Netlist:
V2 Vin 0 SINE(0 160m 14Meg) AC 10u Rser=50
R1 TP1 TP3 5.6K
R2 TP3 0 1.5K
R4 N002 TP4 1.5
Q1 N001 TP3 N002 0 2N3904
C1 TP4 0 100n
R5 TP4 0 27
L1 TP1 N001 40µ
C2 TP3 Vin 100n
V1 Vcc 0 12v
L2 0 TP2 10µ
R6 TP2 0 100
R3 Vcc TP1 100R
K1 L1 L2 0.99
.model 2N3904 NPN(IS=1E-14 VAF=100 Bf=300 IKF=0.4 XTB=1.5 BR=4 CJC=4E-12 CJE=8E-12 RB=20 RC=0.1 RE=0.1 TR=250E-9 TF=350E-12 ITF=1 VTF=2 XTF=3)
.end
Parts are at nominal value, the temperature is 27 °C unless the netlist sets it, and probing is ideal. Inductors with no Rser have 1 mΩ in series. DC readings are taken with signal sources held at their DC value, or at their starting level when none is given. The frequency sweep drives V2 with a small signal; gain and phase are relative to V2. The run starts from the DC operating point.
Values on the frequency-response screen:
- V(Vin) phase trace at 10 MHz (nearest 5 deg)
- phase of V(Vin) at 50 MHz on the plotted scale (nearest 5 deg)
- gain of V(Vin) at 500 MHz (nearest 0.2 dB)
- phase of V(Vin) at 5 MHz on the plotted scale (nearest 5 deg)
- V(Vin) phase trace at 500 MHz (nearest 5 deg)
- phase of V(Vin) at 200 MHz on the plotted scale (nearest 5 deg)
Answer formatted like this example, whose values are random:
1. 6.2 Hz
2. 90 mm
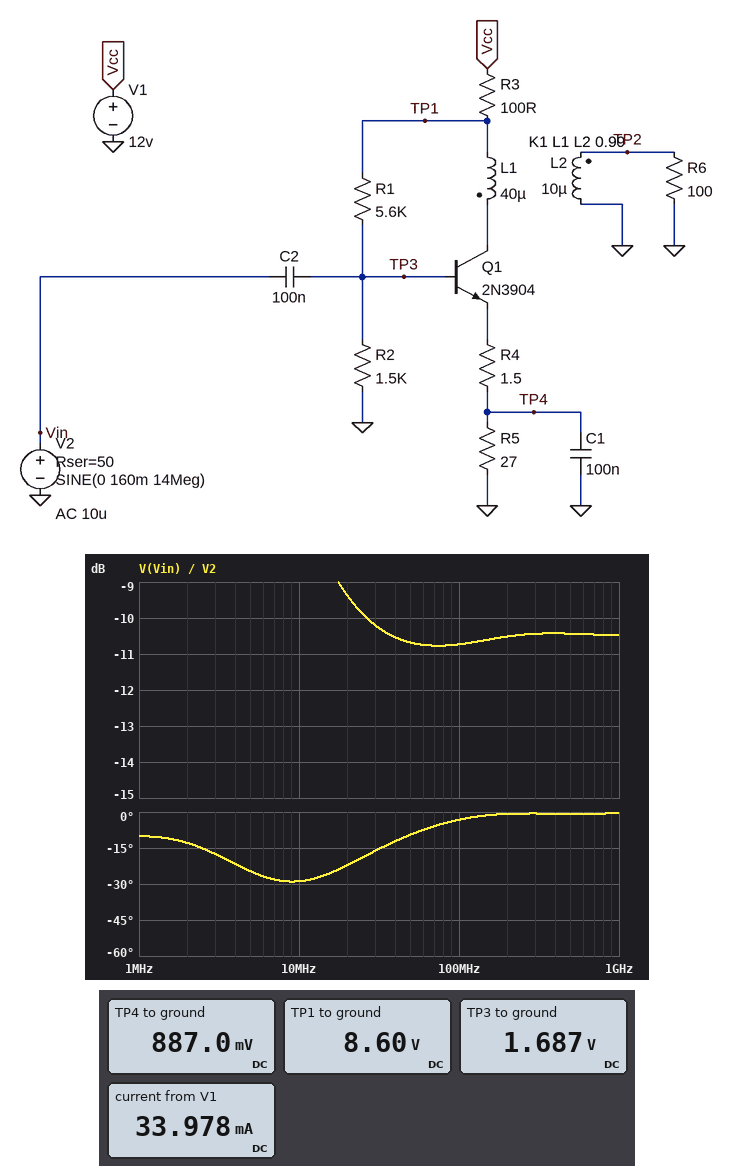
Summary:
1. -30 deg
2. -10 deg
3. -10.4 dB
4. -25 deg
5. 0 deg
6. 0 deg
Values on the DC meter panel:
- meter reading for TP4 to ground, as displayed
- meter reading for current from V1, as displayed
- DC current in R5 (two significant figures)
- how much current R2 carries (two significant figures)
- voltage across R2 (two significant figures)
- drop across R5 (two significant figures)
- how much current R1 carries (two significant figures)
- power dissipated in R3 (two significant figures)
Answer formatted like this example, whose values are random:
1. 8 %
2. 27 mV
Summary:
1. 887.0 mV
2. 33.978 mA
3. 33 mA
4. 1.1 mA
5. 1.7 V
6. 890 mV
7. 1.2 mA
8. 120 mW
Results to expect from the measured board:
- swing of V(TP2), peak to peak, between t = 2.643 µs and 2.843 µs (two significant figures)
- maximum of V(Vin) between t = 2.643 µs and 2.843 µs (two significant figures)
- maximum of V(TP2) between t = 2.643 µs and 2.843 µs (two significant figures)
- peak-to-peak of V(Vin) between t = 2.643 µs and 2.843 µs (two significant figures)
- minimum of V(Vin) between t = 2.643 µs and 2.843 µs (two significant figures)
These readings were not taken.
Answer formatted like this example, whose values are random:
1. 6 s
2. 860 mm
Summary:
1. 6.7 V
2. 61 mV
3. 3.8 V
4. 120 mV
5. -63 mV
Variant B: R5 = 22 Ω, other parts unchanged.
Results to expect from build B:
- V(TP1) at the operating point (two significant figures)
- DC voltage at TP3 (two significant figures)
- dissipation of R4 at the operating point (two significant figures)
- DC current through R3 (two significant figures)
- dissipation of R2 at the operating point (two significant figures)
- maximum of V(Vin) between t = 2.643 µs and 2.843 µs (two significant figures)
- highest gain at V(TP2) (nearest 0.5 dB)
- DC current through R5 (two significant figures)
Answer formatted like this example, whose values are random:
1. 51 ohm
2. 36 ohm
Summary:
1. 8.3 V
2. 1.6 V
3. 2.0 mW
4. 37 mA
5. 1.7 mW
6. 60 mV
7. 34.0 dB
8. 36 mA
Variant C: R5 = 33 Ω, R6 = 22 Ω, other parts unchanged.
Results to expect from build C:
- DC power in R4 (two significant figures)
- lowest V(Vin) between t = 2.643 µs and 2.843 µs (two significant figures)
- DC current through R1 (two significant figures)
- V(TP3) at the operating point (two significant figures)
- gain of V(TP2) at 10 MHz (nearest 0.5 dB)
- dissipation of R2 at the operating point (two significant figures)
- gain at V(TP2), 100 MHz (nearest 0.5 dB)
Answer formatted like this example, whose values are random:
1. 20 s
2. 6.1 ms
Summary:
1. 1.3 mW
2. -110 mV
3. 1.3 mA
4. 1.8 V
5. 19.5 dB
6. 2.1 mW
7. -1.0 dB
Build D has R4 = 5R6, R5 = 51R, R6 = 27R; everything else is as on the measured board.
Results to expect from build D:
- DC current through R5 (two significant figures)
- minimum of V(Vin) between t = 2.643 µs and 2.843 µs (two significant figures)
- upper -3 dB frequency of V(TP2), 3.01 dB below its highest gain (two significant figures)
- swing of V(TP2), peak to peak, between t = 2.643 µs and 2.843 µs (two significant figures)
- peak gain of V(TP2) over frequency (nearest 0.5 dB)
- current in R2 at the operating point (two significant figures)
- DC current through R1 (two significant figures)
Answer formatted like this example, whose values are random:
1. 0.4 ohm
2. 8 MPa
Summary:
1. 22 mA
2. -130 mV
3. 33 MHz
4. 1.8 V
5. 16.0 dB
6. 1.3 mA
7. 1.4 mA
